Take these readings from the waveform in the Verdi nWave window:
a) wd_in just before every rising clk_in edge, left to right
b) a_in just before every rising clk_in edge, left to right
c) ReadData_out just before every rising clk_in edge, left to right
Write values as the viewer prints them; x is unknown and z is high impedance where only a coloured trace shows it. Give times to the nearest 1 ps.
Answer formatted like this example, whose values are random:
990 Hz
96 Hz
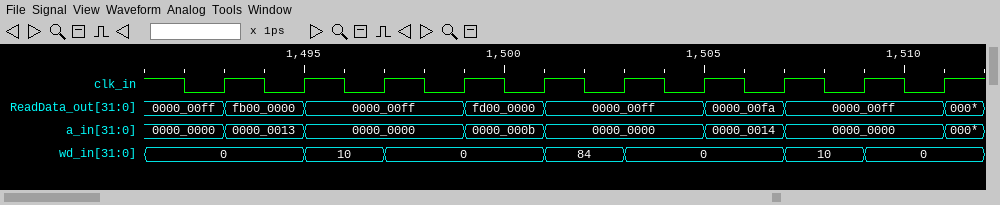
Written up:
0, 0, 10, 0, 0, 84, 0, 0, 10, 0
0000_0000, 0000_0013, 0000_0000, 0000_0000, 0000_000b, 0000_0000, 0000_0000, 0000_0014, 0000_0000, 0000_0000
0000_00ff, fb00_0000, 0000_00ff, 0000_00ff, fd00_0000, 0000_00ff, 0000_00ff, 0000_00fa, 0000_00ff, 0000_00ff
